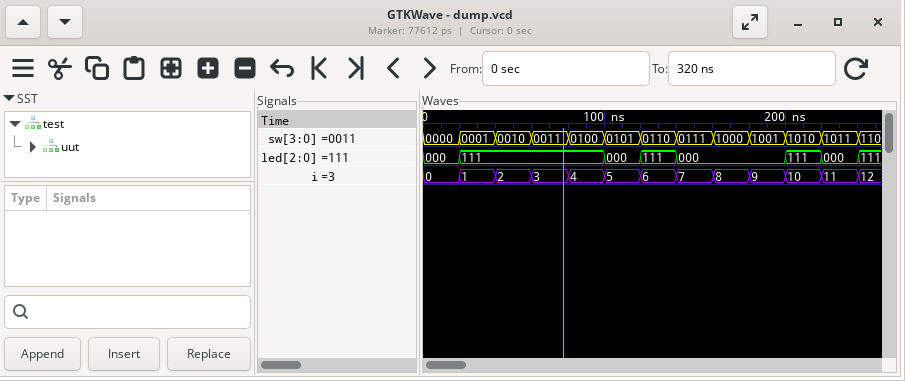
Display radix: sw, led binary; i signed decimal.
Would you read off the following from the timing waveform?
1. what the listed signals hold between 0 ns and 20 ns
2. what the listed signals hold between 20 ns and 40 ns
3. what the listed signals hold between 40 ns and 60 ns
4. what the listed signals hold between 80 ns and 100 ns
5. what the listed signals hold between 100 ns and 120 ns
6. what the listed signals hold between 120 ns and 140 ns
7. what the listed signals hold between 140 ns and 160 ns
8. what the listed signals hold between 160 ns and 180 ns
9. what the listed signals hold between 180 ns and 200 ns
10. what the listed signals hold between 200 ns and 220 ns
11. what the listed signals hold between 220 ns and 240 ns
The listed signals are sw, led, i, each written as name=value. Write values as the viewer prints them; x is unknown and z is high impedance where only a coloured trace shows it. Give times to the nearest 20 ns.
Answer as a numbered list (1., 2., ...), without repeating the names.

1. sw=0000, led=000, i=0
2. sw=0001, led=111, i=1
3. sw=0010, led=111, i=2
4. sw=0100, led=111, i=4
5. sw=0101, led=000, i=5
6. sw=0110, led=111, i=6
7. sw=0111, led=000, i=7
8. sw=1000, led=000, i=8
9. sw=1001, led=000, i=9
10. sw=1010, led=111, i=10
11. sw=1011, led=000, i=11
